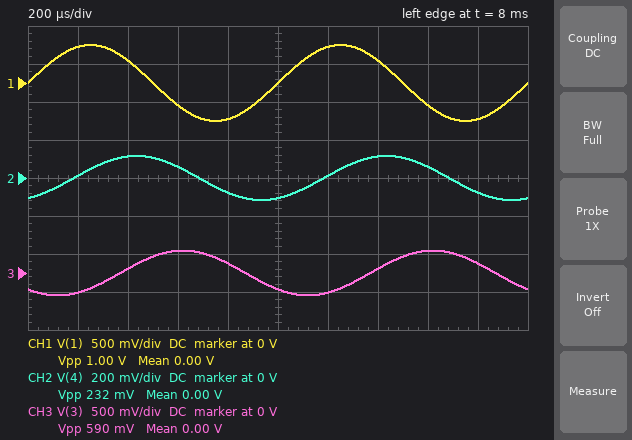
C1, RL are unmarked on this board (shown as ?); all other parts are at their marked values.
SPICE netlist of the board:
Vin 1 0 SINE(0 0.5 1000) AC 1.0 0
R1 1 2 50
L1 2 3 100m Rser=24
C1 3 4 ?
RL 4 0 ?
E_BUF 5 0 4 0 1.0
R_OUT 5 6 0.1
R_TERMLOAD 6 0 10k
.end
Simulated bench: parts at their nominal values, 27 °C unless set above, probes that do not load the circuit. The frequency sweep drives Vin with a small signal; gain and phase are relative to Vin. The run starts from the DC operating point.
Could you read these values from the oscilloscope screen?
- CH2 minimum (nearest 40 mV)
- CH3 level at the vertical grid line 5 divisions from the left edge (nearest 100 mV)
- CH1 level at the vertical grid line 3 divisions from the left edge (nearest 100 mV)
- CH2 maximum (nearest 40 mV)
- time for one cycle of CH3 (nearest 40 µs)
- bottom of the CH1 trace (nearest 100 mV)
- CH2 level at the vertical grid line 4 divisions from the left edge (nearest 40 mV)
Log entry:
-120 mV
-200 mV
-300 mV
120 mV
1.00 ms
-500 mV
-80 mV
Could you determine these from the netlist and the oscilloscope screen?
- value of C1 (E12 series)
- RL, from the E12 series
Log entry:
680 nF
100 Ω
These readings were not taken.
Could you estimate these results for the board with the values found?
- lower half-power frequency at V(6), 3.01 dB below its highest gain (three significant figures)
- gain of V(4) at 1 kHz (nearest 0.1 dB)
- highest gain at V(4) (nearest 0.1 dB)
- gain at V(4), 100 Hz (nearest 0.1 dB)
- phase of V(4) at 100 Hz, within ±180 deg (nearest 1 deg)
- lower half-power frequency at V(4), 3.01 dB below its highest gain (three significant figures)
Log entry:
487 Hz
-12.7 dB
-4.8 dB
-27.2 dB
86 deg
487 Hz
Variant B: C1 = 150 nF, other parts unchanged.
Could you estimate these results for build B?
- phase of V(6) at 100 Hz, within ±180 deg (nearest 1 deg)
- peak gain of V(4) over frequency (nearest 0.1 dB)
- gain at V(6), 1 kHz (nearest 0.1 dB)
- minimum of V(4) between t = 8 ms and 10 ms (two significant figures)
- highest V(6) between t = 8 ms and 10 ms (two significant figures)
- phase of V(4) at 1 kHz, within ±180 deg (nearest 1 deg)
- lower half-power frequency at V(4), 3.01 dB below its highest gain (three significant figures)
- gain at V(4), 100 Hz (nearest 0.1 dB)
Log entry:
89 deg
-4.8 dB
-13.4 dB
-110 mV
110 mV
68 deg
1.17 kHz
-40.5 dB
